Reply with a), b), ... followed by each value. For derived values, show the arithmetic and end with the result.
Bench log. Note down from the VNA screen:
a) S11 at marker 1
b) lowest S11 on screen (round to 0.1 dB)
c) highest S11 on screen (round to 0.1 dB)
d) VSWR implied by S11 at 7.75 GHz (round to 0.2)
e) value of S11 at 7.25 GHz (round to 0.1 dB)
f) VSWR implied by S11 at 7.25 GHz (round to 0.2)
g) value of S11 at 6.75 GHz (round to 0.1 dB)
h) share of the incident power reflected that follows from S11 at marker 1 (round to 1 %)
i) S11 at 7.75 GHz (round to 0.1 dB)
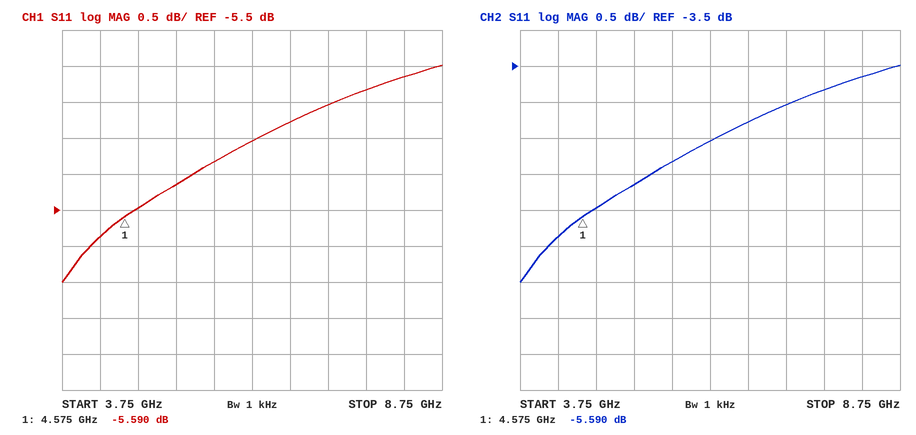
a) -5.590 dB
b) -6.5 dB
c) -3.5 dB
d) |Γ| = 10^(-3.8/20) = 0.6457; VSWR = (1 + 0.6457)/(1 − 0.6457) ≈ 4.6
e) -4.0 dB
f) |Γ| = 10^(-4/20) = 0.6310; VSWR = (1 + 0.6310)/(1 − 0.6310) ≈ 4.4
g) -4.3 dB
h) 10^(-5.59/10) ≈ 28 %
i) -3.8 dB
